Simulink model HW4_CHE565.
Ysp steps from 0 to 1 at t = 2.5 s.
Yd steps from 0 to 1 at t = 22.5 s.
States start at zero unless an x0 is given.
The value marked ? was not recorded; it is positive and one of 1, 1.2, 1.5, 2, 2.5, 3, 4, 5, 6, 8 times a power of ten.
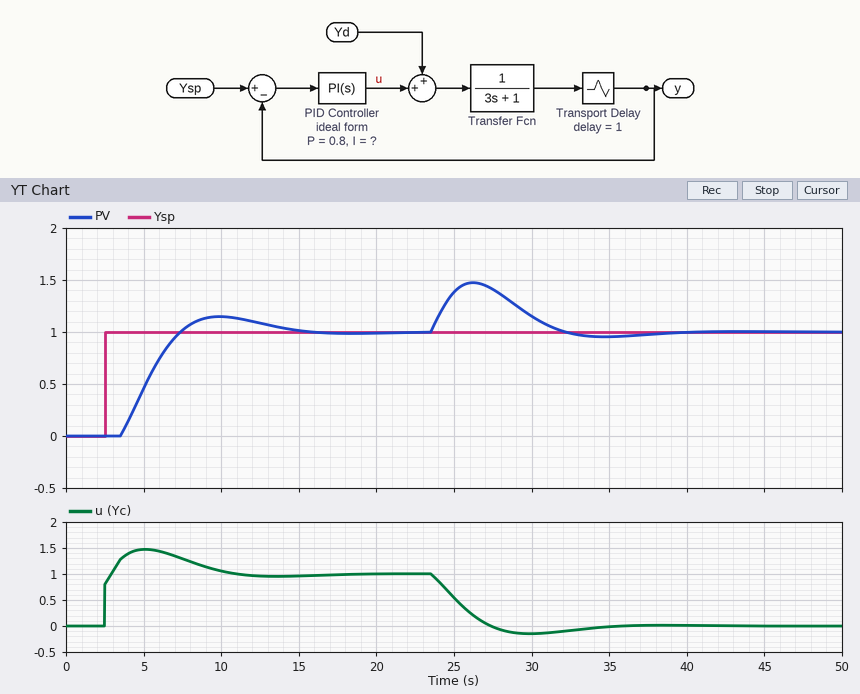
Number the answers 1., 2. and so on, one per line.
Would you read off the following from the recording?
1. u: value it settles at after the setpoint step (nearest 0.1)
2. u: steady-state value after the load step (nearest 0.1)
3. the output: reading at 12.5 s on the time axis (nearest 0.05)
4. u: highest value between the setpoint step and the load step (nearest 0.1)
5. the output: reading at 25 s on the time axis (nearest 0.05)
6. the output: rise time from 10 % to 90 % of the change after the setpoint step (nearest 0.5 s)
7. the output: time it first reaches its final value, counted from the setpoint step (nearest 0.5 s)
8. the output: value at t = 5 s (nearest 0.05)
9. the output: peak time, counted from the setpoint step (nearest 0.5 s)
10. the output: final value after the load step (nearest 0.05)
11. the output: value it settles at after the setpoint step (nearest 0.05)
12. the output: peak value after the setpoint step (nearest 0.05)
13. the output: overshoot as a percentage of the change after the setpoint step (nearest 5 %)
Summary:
1. 1.0
2. 0.0
3. 1.10
4. 1.5
5. 1.40
6. 3.0 s
7. 5.0 s
8. 0.45
9. 7.5 s
10. 1.00
11. 1.00
12. 1.15
13. 15 %
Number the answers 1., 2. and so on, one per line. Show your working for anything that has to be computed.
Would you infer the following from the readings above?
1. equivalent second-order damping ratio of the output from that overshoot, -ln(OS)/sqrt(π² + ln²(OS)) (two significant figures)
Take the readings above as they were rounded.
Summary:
1. ln(0.15) = -1.897; 1.897 / sqrt(9.870 + 3.599) = 0.52
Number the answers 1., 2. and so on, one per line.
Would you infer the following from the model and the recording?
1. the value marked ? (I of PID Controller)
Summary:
1. 0.6
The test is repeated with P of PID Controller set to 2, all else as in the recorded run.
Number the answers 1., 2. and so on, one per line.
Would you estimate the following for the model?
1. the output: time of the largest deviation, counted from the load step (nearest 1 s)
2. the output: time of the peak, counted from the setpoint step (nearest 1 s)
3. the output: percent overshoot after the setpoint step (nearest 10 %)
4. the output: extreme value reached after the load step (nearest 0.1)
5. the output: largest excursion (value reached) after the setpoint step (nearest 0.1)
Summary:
1. 3 s
2. 4 s
3. 50 %
4. 1.4
5. 1.5
